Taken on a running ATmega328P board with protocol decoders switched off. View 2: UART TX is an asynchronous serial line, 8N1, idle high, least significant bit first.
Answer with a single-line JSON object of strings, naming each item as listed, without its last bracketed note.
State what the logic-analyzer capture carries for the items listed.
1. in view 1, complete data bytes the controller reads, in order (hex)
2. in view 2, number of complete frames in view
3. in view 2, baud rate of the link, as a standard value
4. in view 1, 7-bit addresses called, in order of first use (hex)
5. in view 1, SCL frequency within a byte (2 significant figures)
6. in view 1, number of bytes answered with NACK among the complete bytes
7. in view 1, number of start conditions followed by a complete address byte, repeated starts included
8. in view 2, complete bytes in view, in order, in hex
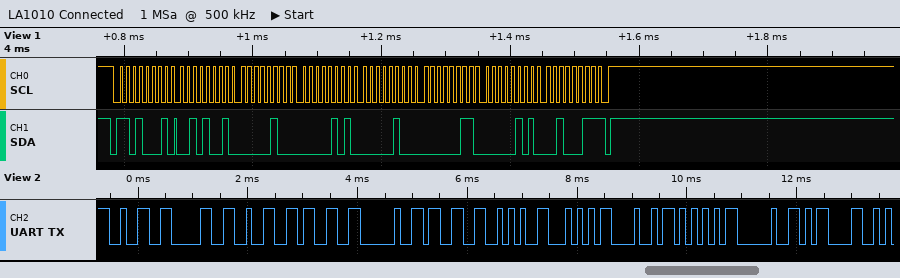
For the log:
{"in view 1, complete data bytes the controller reads, in order": "29 04 05 04 03 05 23", "in view 2, number of complete frames in view": "12", "in view 2, baud rate of the link, as a standard value": "9600 baud", "in view 1, 7-bit addresses called, in order of first use": "0x68", "in view 1, SCL frequency within a byte": "100 kHz", "in view 1, number of bytes answered with NACK among the complete bytes": "1", "in view 1, number of start conditions followed by a complete address byte, repeated starts included": "1", "in view 2, complete bytes in view, in order, in hex": "0x32 0x30 0x32 0x33 0x20 0x33 0x2A 0x54 0x48 0x55 0x20 0x0D"}
